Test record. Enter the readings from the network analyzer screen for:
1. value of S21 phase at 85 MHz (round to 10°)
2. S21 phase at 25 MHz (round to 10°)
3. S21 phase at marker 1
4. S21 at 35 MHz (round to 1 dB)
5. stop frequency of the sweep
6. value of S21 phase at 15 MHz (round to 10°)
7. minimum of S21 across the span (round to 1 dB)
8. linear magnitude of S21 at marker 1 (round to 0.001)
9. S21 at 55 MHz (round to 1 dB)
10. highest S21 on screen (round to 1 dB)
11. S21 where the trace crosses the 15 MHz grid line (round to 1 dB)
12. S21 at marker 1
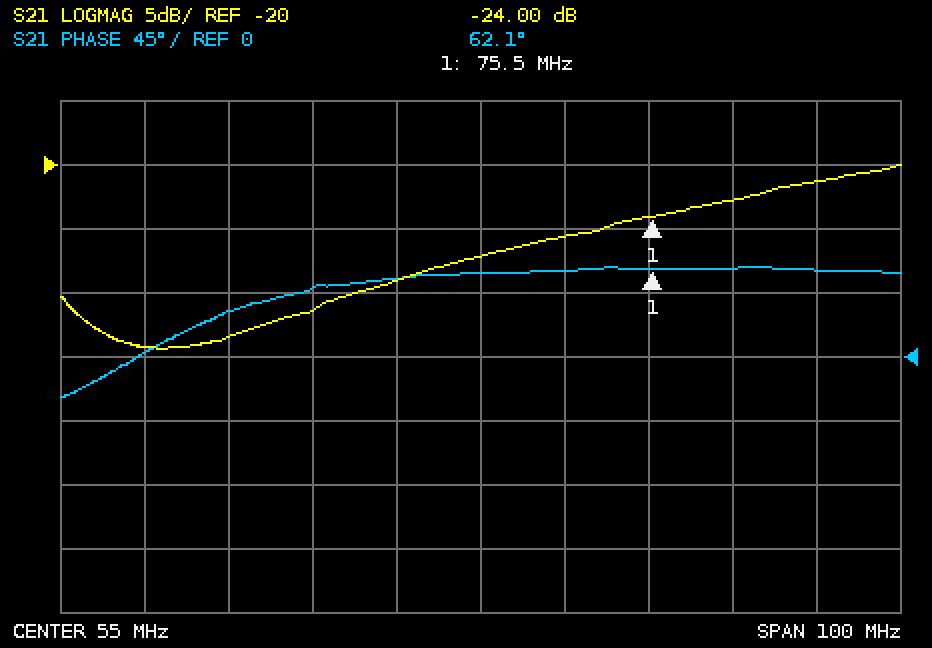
60°
30°
62.1°
-31 dB
105 MHz
0°
-34 dB
0.063
-27 dB
-20 dB
-34 dB
-24.00 dB
